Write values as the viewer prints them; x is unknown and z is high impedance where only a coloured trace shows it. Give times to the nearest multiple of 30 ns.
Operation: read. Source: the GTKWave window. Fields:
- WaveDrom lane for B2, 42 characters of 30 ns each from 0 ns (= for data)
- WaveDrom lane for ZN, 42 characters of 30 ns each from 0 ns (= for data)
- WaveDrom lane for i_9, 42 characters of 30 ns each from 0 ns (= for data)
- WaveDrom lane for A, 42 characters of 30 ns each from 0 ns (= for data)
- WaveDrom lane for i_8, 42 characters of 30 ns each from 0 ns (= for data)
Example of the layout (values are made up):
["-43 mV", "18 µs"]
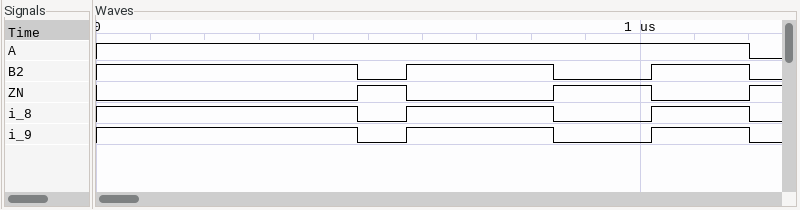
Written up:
["{name: 'B2', wave: '1...............0..1........0.....1.....0.'}", "{name: 'ZN', wave: '0...............1..0........1.....0.....1.'}", "{name: 'i_9', wave: '1...............0..1........0.....1.....0.'}", "{name: 'A', wave: '1.......................................0.'}", "{name: 'i_8', wave: '1...............0..1........0.....1.....0.'}"]
